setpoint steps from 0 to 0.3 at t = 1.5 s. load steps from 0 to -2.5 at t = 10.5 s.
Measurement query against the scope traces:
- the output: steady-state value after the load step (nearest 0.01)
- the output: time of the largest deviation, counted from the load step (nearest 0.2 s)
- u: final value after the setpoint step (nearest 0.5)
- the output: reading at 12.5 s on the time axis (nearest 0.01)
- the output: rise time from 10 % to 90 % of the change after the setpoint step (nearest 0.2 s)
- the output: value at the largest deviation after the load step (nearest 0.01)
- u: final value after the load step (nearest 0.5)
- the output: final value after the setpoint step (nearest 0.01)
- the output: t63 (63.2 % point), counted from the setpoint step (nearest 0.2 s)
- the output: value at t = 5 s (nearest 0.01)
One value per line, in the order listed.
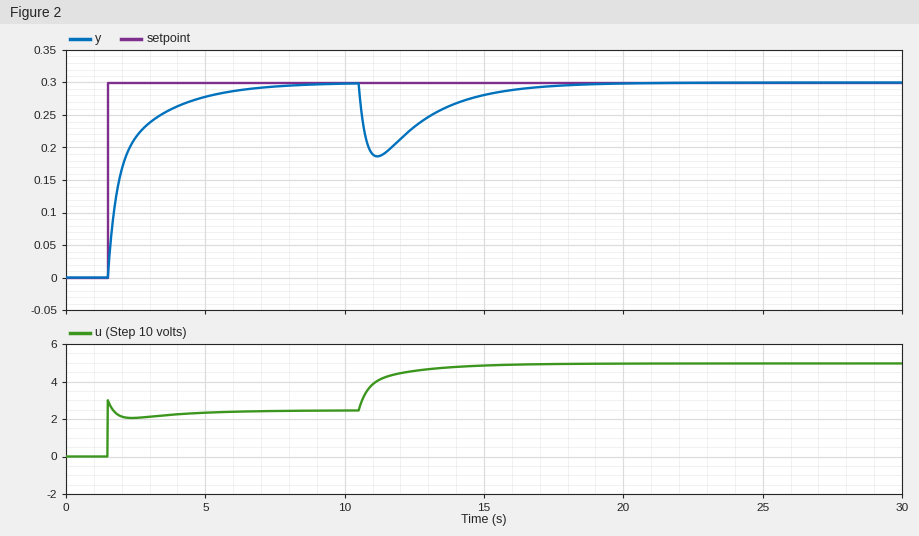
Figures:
0.30
0.6 s
2.5
0.23
2.8 s
0.19
5.0
0.30
0.6 s
0.28
